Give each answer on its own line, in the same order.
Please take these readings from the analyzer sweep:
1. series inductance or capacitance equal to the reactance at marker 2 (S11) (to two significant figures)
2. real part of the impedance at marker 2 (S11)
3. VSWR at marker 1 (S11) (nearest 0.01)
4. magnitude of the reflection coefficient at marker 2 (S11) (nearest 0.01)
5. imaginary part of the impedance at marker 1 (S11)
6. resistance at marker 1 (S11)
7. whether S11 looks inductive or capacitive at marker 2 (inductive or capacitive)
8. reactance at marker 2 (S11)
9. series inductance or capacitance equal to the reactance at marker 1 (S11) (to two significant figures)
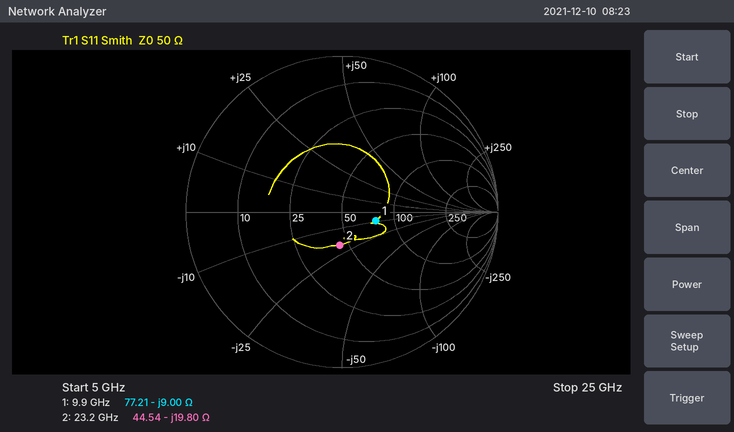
350 fF
44.54 Ω
1.58
0.21
-9.00 Ω
77.21 Ω
capacitive
-19.80 Ω
1.8 pF
